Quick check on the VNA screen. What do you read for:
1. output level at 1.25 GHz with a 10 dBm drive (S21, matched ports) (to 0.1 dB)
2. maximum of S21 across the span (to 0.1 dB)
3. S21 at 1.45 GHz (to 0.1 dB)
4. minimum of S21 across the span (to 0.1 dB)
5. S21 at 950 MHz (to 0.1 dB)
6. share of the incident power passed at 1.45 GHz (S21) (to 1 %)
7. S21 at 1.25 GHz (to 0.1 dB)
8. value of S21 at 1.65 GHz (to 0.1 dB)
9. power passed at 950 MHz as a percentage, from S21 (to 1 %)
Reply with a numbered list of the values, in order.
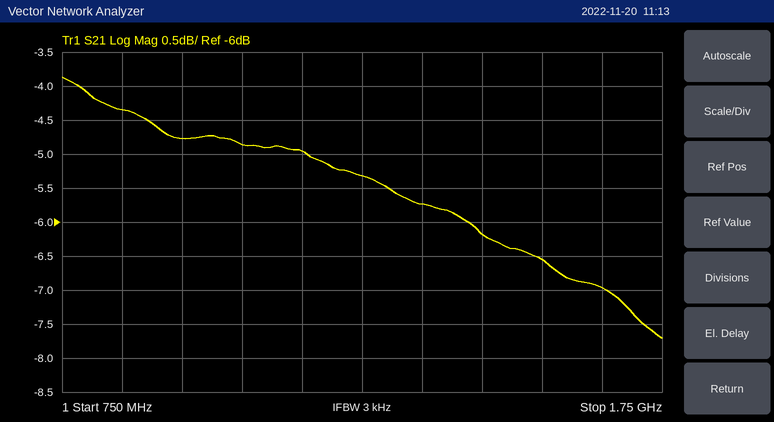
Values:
1. 4.7 dBm
2. -3.9 dB
3. -6.2 dB
4. -7.7 dB
5. -4.8 dB
6. 24 %
7. -5.3 dB
8. -7.0 dB
9. 33 %
